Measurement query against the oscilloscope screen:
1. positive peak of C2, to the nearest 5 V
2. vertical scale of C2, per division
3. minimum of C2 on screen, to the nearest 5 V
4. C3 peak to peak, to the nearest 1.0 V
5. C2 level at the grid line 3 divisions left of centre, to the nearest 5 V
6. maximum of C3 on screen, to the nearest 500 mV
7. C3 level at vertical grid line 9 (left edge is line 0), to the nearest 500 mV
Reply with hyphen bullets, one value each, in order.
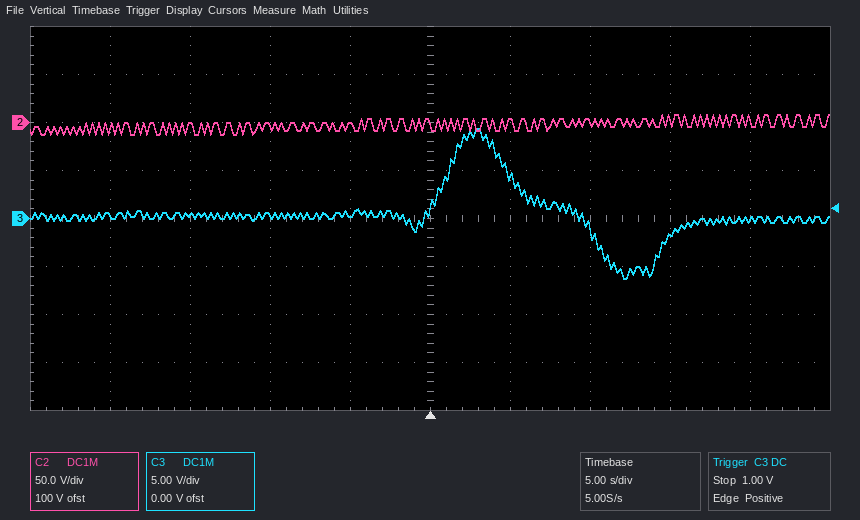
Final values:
- 10 V
- 50 V
- -10 V
- 16.0 V
- -5 V
- 9.5 V
- 0.0 V
